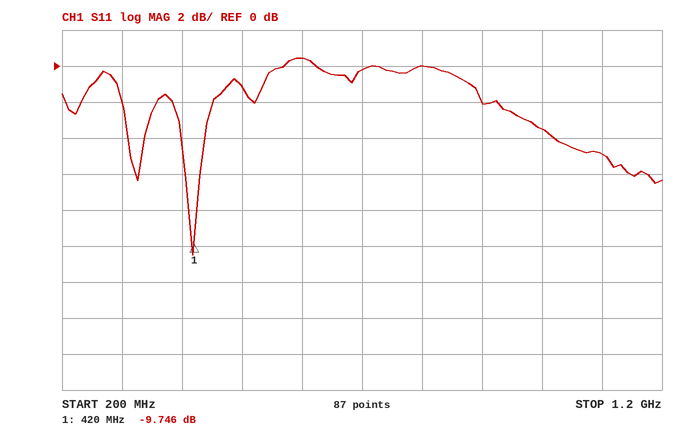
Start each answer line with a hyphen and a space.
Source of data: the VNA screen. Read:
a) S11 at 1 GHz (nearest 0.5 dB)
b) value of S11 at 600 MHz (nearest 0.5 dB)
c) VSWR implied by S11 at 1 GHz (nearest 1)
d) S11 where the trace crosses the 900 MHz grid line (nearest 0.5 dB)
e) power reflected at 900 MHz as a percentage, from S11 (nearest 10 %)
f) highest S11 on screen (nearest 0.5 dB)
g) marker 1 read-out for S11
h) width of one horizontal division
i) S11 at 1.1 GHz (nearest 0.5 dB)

- -3.5 dB
- 0.5 dB
- 5
- -2.0 dB
- 60 %
- 0.5 dB
- -9.746 dB
- 100 MHz
- -5.0 dB
